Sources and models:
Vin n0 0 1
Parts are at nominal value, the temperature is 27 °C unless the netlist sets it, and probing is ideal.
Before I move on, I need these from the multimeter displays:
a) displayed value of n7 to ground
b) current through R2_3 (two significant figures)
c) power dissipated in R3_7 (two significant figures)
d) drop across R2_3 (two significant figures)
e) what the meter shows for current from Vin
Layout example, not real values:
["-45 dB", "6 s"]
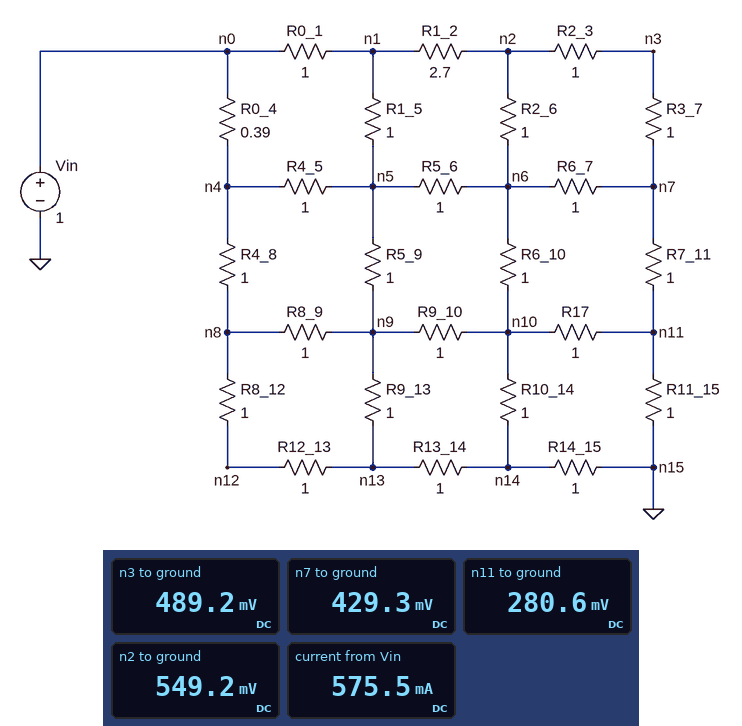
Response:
["429.3 mV", "60 mA", "3.6 mW", "60 mV", "575.5 mA"]
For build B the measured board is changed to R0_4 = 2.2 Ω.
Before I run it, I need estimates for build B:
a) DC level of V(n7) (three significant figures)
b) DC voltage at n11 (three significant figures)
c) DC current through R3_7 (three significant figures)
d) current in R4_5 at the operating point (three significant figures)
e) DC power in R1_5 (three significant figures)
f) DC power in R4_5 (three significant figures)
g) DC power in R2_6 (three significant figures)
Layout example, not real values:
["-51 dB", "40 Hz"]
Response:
["352 mV", "226 mV", "55.6 mA", "60.2 mA", "32.0 mW", "3.62 mW", "1.70 mW"]
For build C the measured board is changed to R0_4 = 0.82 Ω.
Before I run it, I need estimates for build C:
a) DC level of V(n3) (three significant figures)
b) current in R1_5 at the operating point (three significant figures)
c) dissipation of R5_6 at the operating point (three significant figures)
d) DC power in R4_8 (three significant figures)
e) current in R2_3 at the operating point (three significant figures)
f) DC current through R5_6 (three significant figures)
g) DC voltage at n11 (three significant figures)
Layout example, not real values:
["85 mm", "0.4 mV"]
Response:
["457 mV", "139 mA", "21.8 mW", "27.6 mW", "58.2 mA", "148 mA", "259 mV"]
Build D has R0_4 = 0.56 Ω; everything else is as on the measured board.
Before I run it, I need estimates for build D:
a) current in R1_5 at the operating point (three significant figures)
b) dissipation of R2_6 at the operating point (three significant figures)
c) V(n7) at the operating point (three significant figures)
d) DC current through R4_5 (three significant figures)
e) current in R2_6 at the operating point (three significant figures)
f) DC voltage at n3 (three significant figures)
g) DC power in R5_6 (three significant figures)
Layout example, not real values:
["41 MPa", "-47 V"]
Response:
["125 mA", "1.08 mW", "416 mV", "154 mA", "32.9 mA", "475 mV", "24.4 mW"]
